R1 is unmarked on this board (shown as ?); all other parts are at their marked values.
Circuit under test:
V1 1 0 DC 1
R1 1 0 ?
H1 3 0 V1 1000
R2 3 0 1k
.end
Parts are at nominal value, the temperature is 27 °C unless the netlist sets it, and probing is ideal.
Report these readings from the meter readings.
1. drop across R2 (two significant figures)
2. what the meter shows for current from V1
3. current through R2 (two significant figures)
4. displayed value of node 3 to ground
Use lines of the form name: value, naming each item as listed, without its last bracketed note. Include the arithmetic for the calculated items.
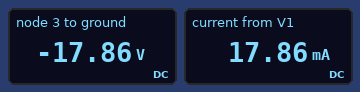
drop across R2: 0 V - (-17.86 V) = 18 V
what the meter shows for current from V1: 17.86 mA
current through R2: (0 V - (-17.86 V)) / 1 kΩ = 18 mA
displayed value of node 3 to ground: -17.86 V
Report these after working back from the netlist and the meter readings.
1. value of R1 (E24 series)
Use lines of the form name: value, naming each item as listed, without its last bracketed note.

value of R1: 56 Ω
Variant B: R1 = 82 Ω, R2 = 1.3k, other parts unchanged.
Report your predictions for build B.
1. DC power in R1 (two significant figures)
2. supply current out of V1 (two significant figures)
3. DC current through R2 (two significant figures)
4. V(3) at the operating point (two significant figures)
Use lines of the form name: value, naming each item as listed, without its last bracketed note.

DC power in R1: 12 mW
supply current out of V1: 12 mA
DC current through R2: 9.4 mA
V(3) at the operating point: -12 V
